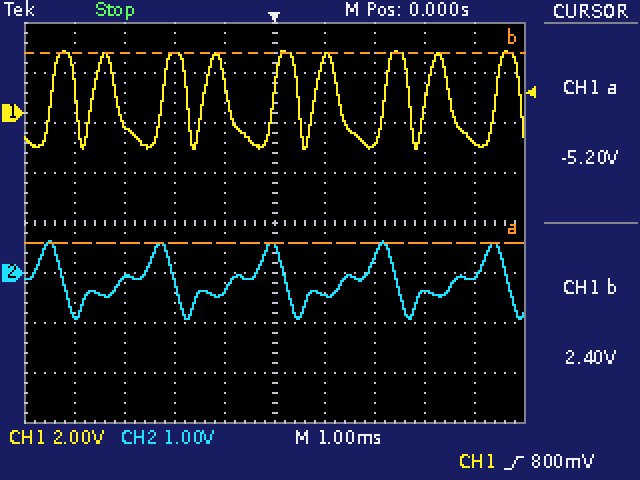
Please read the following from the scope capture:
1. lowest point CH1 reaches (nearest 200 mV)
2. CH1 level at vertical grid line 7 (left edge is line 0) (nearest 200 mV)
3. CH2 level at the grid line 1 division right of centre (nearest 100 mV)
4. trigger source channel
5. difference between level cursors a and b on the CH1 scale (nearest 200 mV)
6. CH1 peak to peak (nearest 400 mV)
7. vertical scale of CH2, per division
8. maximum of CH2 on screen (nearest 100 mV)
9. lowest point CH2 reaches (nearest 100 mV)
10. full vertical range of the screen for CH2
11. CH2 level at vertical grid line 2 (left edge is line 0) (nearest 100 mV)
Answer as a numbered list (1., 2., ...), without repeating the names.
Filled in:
1. -1.4 V
2. -1.2 V
3. -400 mV
4. CH1
5. 7.6 V
6. 4.0 V
7. 1 V
8. 600 mV
9. -900 mV
10. 8 V
11. -100 mV
